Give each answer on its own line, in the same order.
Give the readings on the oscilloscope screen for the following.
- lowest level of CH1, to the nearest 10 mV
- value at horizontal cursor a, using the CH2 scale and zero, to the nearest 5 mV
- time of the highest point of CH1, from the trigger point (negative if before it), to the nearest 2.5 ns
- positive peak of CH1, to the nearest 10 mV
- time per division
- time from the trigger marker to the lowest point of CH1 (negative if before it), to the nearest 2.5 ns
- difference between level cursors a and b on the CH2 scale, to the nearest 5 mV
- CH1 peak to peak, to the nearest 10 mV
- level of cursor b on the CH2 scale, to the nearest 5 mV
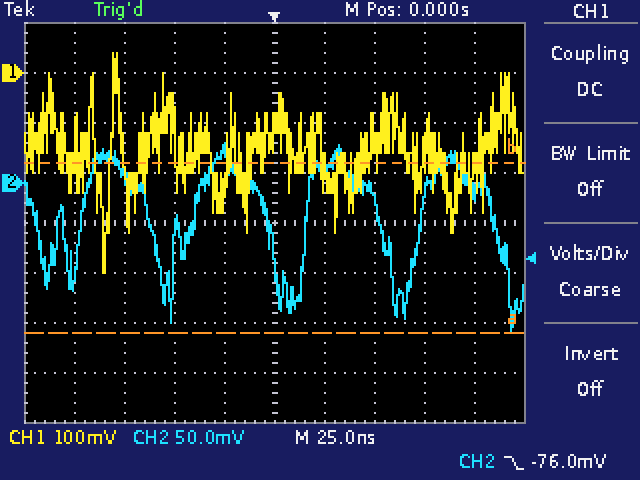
-400 mV
-150 mV
-80.0 ns
40 mV
25 ns
-85.0 ns
170 mV
440 mV
20 mV
